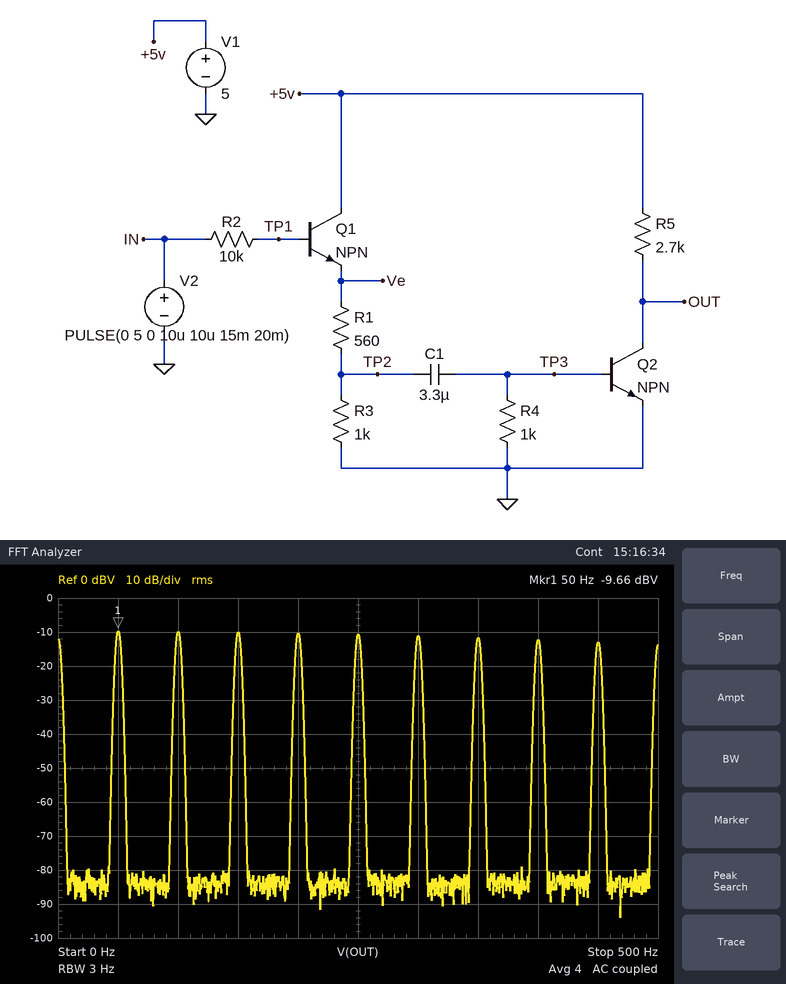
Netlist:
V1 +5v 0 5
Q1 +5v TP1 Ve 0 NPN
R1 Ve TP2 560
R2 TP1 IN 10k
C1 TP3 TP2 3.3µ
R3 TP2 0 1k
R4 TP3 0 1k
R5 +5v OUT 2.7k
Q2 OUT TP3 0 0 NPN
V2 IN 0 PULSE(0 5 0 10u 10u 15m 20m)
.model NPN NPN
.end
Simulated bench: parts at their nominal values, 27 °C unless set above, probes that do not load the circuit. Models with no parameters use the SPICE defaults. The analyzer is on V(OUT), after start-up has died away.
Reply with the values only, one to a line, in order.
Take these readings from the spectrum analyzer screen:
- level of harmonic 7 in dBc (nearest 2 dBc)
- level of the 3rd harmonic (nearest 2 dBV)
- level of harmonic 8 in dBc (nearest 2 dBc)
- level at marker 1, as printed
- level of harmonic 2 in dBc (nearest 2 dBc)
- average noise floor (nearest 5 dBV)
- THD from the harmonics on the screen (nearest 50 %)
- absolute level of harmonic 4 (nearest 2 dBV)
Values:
-2 dBc
-10 dBV
-2 dBc
-9.66 dBV
0 dBc
-85 dBV
250 %
-10 dBV
